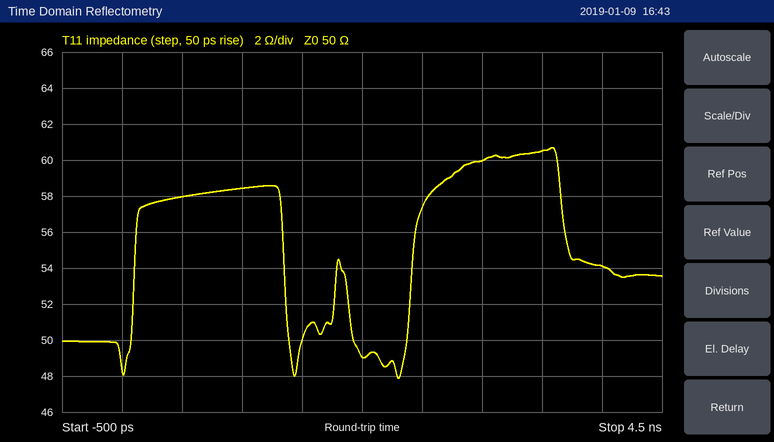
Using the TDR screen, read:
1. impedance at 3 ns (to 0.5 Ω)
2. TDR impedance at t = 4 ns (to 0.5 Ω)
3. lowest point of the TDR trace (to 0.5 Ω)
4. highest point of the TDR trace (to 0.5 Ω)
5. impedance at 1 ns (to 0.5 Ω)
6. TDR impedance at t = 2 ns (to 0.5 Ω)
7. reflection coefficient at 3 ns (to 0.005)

60.0 Ω
54.0 Ω
48.0 Ω
60.5 Ω
58.5 Ω
49.0 Ω
+0.090
